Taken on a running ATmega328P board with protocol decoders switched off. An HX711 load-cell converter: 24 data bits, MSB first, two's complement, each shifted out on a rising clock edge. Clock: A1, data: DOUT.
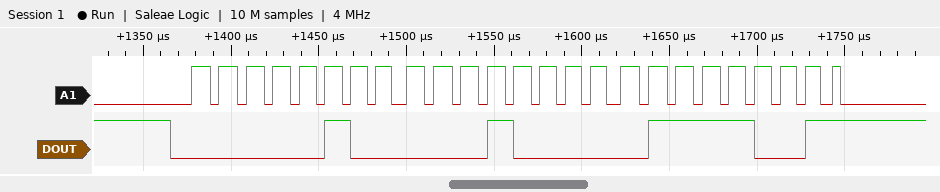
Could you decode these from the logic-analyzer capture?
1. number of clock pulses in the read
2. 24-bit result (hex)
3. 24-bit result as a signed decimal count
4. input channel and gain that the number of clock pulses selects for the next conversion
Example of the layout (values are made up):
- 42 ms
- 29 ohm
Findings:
- 25
- 0x041079
- 266361
- channel A, gain 128
